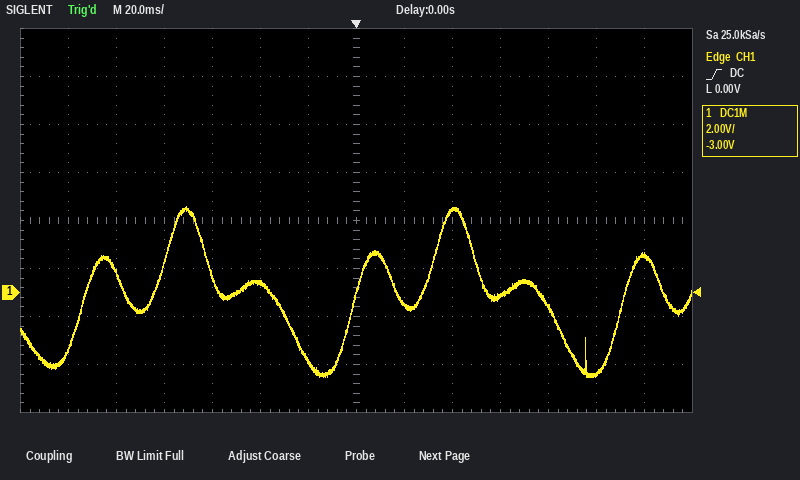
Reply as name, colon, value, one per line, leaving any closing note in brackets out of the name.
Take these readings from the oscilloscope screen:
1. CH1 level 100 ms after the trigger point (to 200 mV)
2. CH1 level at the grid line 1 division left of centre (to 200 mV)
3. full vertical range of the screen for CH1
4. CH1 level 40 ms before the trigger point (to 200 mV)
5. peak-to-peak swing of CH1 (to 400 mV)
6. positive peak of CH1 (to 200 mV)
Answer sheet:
CH1 level 100 ms after the trigger point: -3.4 V
CH1 level at the grid line 1 division left of centre: -2.8 V
full vertical range of the screen for CH1: 16 V
CH1 level 40 ms before the trigger point: 400 mV
peak-to-peak swing of CH1: 7.2 V
positive peak of CH1: 3.6 V
